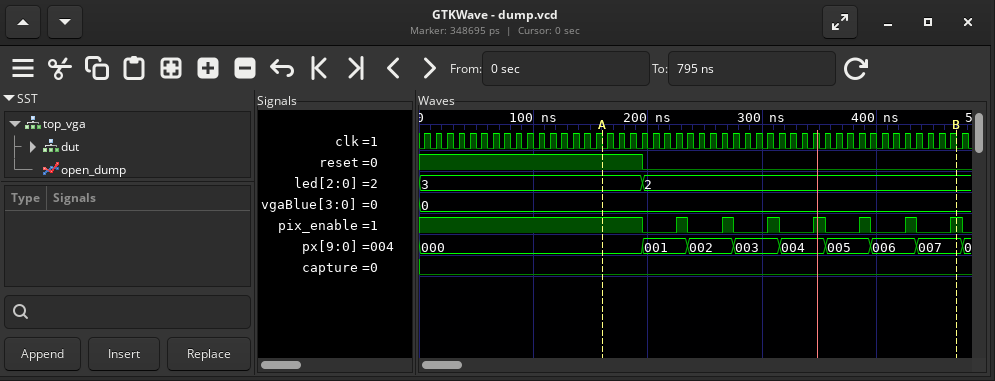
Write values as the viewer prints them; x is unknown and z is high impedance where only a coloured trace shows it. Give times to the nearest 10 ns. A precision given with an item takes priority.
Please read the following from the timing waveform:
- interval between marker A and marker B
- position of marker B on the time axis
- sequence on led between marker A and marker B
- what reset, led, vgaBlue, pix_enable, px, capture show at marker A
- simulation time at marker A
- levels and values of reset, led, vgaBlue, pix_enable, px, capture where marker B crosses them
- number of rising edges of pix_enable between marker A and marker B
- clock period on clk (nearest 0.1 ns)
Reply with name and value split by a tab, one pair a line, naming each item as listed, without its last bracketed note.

interval between marker A and marker B	310 ns
position of marker B on the time axis	470 ns
sequence on led between marker A and marker B	3, 2
what reset, led, vgaBlue, pix_enable, px, capture show at marker A	reset=1, led=3, vgaBlue=0, pix_enable=1, px=000, capture=0
simulation time at marker A	160 ns
levels and values of reset, led, vgaBlue, pix_enable, px, capture where marker B crosses them	reset=0, led=2, vgaBlue=0, pix_enable=1, px=007, capture=0
number of rising edges of pix_enable between marker A and marker B	7
clock period on clk	10 ns
